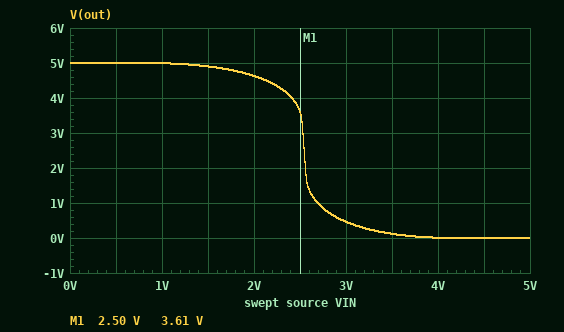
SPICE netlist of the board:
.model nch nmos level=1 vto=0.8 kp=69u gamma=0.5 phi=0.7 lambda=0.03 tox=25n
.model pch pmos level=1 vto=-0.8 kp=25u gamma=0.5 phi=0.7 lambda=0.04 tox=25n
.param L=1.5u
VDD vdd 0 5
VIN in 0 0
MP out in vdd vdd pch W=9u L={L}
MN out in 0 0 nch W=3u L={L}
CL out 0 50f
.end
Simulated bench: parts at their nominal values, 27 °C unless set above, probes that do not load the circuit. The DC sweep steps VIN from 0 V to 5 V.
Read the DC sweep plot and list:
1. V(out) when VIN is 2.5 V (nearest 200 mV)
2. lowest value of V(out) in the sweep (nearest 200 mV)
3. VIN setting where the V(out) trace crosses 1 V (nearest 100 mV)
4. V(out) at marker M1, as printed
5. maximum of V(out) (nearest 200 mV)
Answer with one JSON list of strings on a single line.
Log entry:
["3.6 V", "0 V", "2.7 V", "3.61 V", "5.0 V"]
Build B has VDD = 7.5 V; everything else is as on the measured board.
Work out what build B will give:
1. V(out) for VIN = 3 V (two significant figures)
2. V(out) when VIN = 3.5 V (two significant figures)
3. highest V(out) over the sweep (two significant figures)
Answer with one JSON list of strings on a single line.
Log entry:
["6.7 V", "6.0 V", "7.5 V"]
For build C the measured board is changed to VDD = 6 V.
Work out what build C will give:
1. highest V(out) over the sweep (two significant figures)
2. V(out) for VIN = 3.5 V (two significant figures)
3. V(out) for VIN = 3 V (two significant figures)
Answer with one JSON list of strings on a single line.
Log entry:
["6.0 V", "810 mV", "4.2 V"]
